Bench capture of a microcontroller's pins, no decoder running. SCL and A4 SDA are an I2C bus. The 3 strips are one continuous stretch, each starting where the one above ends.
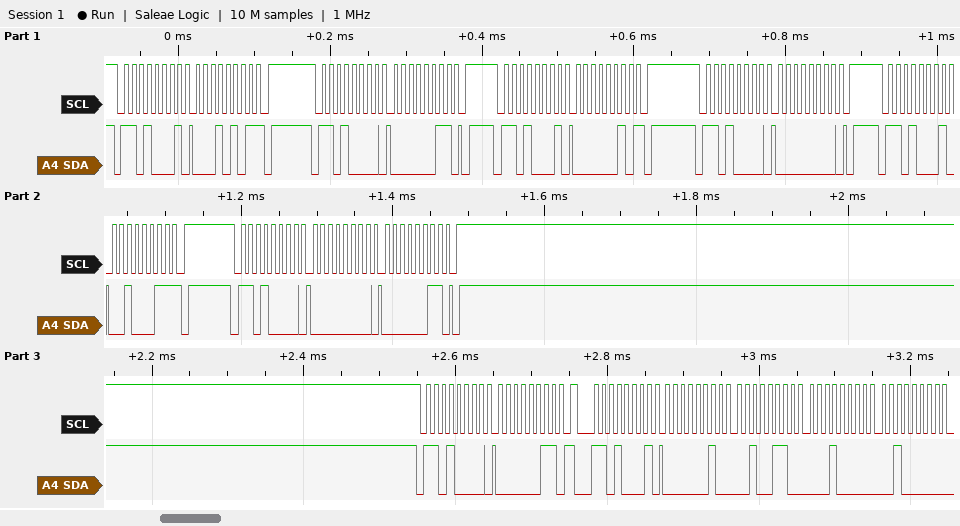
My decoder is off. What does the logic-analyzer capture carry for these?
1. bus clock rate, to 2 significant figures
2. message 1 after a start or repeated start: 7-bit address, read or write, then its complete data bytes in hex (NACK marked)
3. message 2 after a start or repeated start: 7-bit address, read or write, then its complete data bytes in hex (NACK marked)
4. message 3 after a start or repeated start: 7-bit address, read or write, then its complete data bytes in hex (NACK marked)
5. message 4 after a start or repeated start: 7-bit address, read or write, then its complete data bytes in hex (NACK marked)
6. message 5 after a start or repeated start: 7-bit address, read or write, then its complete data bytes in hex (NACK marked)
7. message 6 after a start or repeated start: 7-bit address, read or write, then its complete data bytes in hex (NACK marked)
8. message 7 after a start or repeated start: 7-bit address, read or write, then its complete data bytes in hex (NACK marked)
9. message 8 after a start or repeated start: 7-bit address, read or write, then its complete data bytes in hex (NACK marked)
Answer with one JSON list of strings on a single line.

["100 kHz", "0x68 read: 15 NACK", "0x68 write: 03", "0x68 read: 02 NACK", "0x68 write: 00", "0x68 read: 23 NACK", "0x68 write: 00 03", "0x68 write: 03", "0x68 read: 02 26 10 20"]
